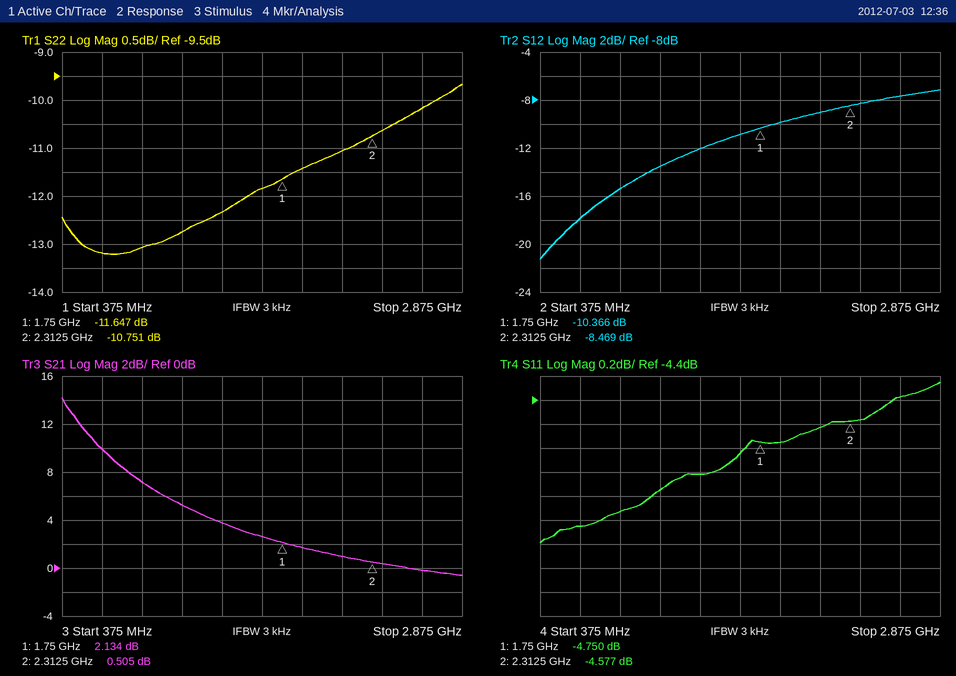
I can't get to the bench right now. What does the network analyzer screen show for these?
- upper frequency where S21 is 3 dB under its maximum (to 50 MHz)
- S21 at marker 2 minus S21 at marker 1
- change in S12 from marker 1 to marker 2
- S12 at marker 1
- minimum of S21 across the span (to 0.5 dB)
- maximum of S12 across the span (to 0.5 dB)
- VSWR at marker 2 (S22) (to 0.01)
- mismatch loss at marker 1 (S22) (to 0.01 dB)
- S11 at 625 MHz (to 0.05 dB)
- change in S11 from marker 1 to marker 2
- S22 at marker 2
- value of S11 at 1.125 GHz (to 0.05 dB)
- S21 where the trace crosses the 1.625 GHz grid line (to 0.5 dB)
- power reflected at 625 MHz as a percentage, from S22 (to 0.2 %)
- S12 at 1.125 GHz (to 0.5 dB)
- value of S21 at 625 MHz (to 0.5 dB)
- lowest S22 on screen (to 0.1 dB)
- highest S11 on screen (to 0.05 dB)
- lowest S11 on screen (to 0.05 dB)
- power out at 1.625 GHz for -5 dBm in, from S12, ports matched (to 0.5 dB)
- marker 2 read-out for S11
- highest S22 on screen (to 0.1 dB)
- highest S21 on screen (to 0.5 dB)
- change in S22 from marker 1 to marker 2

550 MHz
-1.629 dB
1.897 dB
-10.366 dB
-0.5 dB
-7.0 dB
1.82
0.31 dB
-5.45 dB
0.173 dB
-10.751 dB
-5.15 dB
2.5 dB
4.8 %
-13.5 dB
10.0 dB
-13.2 dB
-4.25 dB
-5.60 dB
-16.0 dBm
-4.577 dB
-9.7 dB
14.0 dB
0.896 dB
